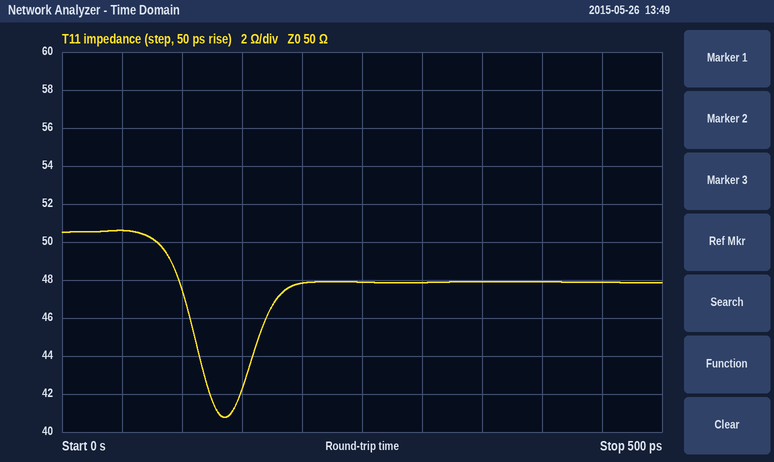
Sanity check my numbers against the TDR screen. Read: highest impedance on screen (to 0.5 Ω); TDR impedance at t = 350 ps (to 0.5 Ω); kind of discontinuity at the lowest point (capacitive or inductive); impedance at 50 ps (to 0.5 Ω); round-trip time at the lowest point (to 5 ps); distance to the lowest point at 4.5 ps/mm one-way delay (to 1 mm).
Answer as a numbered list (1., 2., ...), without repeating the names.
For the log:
1. 50.5 Ω
2. 48.0 Ω
3. capacitive
4. 50.5 Ω
5. 135 ps
6. 15 mm
